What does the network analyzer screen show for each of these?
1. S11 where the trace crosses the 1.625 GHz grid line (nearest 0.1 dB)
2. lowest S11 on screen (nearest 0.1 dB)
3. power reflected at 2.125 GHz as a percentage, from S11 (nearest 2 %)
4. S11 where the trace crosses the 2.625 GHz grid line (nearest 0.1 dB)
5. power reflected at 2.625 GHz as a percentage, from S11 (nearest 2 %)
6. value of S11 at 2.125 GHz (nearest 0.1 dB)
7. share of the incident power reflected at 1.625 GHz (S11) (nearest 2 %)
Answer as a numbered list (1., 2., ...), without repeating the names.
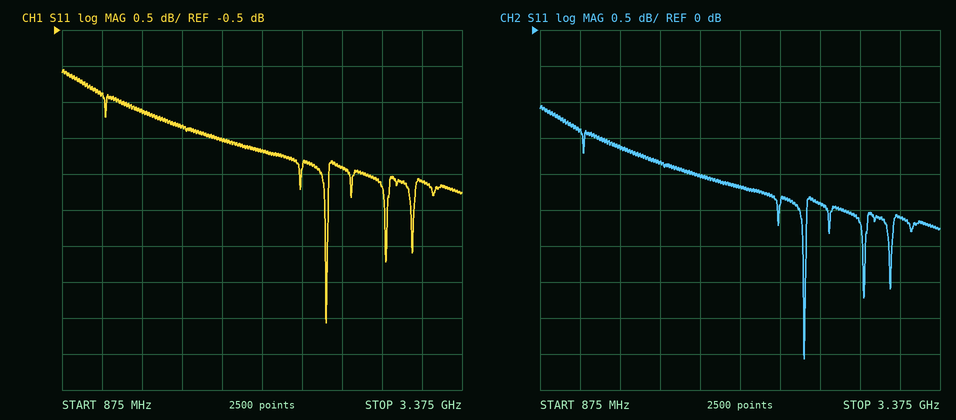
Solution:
1. -1.8 dB
2. -4.6 dB
3. 60 %
4. -2.4 dB
5. 58 %
6. -2.2 dB
7. 66 %
